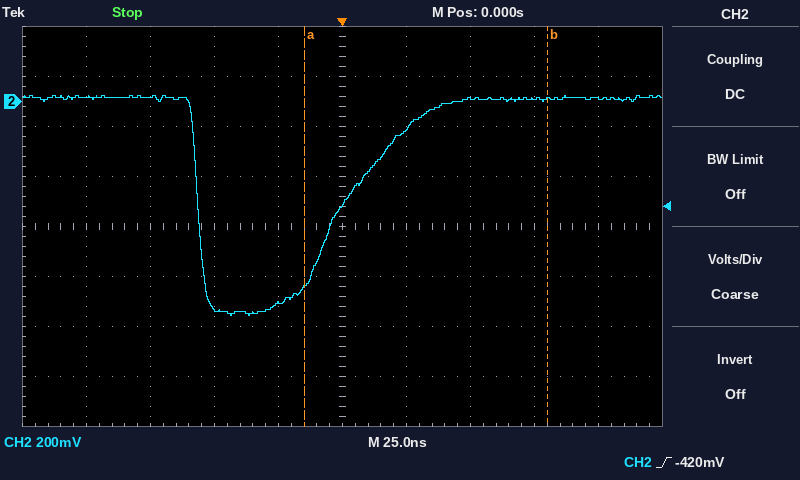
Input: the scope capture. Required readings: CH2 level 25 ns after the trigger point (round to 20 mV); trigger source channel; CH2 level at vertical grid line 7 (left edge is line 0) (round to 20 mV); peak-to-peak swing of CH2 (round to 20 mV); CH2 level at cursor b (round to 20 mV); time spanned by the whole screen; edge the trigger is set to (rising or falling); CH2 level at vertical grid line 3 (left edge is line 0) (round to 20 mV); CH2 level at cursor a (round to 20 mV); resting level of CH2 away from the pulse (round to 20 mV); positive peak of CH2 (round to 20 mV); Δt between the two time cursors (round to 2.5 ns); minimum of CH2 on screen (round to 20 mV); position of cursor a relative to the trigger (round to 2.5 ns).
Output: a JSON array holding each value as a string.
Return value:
["-120 mV", "CH2", "20 mV", "880 mV", "20 mV", "250 ns", "rising", "-820 mV", "-740 mV", "20 mV", "20 mV", "95.0 ns", "-860 mV", "-15.0 ns"]
